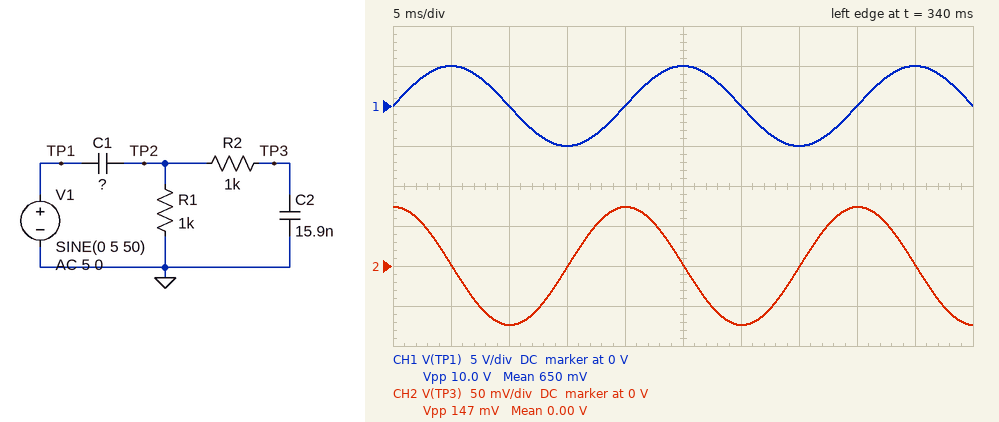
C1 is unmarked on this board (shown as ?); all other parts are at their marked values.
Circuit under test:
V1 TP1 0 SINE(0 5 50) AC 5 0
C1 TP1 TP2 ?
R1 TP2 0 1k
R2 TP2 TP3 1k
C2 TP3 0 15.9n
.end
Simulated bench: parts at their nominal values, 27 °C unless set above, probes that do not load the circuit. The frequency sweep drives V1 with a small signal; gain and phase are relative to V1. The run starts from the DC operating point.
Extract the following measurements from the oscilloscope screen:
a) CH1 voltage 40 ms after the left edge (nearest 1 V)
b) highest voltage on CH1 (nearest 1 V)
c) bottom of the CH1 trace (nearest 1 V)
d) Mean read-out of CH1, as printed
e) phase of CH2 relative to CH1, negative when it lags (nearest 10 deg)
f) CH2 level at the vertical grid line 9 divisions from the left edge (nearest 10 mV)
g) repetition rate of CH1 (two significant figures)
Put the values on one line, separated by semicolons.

0 V; 5 V; -5 V; 650 mV; 90 deg; 0 V; 50 Hz
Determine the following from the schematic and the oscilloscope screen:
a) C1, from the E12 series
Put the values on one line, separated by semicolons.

47 nF
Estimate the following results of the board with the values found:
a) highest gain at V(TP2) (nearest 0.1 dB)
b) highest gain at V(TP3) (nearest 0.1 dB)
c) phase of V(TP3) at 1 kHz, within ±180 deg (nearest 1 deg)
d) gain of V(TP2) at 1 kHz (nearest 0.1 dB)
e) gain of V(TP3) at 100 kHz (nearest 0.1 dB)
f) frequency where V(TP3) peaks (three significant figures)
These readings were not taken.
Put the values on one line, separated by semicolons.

0 dB; -4.5 dB; 63 deg; -11.3 dB; -20.1 dB; 5.82 kHz
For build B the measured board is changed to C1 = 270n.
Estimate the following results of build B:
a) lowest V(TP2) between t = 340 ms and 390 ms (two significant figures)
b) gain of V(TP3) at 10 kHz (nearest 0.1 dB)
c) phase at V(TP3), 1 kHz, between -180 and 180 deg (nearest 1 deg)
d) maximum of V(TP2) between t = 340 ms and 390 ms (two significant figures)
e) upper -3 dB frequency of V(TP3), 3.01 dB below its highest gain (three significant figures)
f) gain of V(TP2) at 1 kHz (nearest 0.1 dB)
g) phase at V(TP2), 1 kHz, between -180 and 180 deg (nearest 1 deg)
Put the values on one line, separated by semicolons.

-420 mV; -3.3 dB; 24 deg; 420 mV; 11.7 kHz; -1.7 dB; 29 deg
